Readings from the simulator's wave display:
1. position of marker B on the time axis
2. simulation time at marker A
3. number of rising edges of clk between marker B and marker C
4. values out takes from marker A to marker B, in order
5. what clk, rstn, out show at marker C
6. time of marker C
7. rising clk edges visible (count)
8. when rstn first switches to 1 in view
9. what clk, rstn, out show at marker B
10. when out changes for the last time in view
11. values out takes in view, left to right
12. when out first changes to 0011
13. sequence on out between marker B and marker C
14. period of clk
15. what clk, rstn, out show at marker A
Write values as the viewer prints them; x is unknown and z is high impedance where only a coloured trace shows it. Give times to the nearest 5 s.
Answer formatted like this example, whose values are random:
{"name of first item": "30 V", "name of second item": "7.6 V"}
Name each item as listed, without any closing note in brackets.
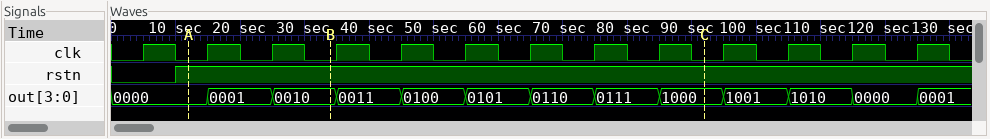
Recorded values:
{"position of marker B on the time axis": "35 s", "simulation time at marker A": "10 s", "number of rising edges of clk between marker B and marker C": "6", "values out takes from marker A to marker B, in order": "0000, 0001, 0010", "what clk, rstn, out show at marker C": "clk=0, rstn=1, out=1000", "time of marker C": "90 s", "rising clk edges visible": "13", "when rstn first switches to 1 in view": "10 s", "what clk, rstn, out show at marker B": "clk=0, rstn=1, out=0010", "when out changes for the last time in view": "125 s", "values out takes in view, left to right": "0000, 0001, 0010, 0011, 0100, 0101, 0110, 0111, 1000, 1001, 1010, 0000, 0001", "when out first changes to 0011": "35 s", "sequence on out between marker B and marker C": "0010, 0011, 0100, 0101, 0110, 0111, 1000", "period of clk": "10 s", "what clk, rstn, out show at marker A": "clk=0, rstn=1, out=0000"}
